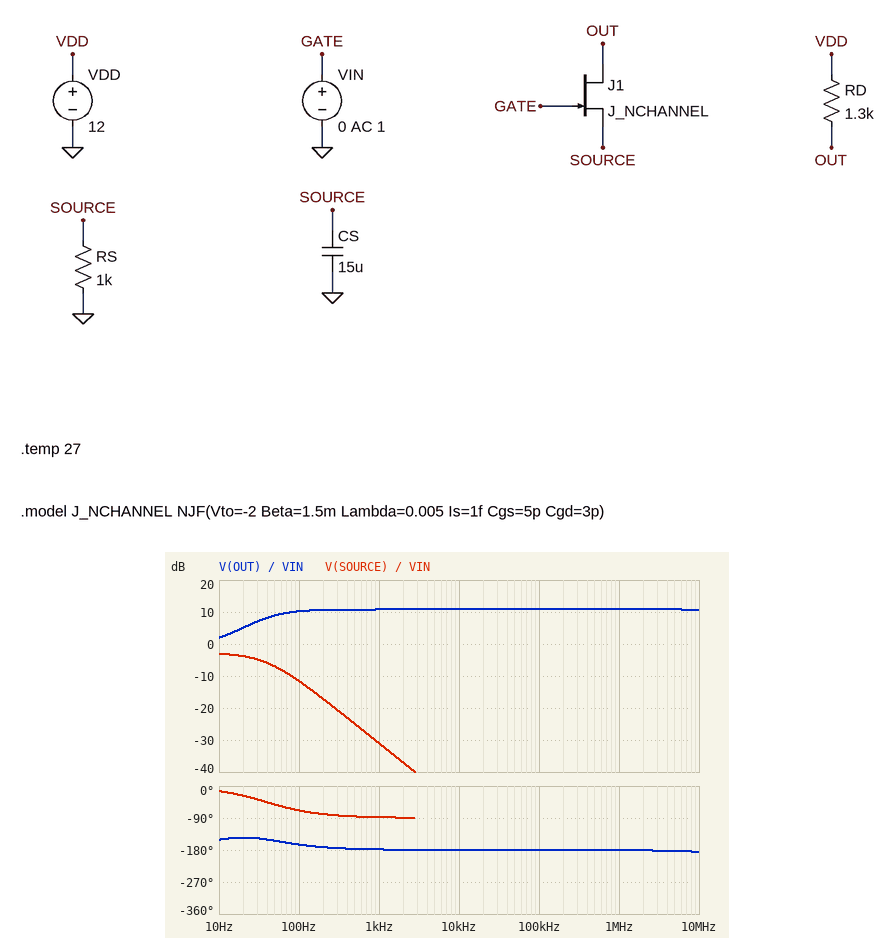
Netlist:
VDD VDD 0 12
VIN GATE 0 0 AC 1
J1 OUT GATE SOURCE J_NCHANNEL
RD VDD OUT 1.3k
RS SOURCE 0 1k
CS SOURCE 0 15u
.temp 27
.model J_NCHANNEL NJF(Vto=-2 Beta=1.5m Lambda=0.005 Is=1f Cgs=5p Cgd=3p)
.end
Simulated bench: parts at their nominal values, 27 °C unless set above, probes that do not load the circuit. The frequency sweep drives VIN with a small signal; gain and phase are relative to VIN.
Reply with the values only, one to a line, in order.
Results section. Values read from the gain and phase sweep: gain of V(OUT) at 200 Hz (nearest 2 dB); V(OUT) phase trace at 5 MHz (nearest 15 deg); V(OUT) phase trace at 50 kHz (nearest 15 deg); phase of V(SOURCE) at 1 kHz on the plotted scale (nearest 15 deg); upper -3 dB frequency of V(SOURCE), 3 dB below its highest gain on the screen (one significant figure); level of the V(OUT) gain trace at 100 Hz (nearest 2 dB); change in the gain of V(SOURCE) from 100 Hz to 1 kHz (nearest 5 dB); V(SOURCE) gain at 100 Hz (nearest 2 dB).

10 dB
-180 deg
-180 deg
-90 deg
40 Hz
10 dB
-20 dB
-12 dB
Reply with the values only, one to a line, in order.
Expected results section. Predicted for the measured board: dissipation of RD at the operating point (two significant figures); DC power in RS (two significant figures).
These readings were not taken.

1.7 mW
1.3 mW
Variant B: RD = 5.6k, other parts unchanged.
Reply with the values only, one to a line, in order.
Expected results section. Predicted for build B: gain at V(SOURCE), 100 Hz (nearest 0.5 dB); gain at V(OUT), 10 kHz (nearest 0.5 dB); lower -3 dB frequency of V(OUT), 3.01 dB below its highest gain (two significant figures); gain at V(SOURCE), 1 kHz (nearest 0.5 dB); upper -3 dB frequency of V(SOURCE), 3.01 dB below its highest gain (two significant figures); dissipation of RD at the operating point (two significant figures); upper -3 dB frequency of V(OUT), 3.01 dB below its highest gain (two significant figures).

-12.0 dB
23.0 dB
35 Hz
-31.5 dB
38 Hz
7.3 mW
25 MHz
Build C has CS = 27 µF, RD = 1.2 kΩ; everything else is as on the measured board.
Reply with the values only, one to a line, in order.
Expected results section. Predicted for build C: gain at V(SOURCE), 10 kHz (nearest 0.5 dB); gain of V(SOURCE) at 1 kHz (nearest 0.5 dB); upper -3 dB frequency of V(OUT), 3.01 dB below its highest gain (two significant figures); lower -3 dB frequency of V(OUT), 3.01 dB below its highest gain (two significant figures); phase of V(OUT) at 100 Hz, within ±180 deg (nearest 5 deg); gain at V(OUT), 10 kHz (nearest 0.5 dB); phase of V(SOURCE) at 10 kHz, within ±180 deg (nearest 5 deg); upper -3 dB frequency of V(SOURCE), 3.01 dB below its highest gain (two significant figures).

-56.0 dB
-36.0 dB
170 MHz
20 Hz
-170 deg
10.0 dB
-90 deg
22 Hz
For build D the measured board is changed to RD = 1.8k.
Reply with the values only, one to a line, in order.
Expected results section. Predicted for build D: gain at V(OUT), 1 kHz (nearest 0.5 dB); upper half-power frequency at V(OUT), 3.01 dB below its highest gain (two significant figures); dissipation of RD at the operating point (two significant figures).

13.5 dB
100 MHz
2.4 mW
